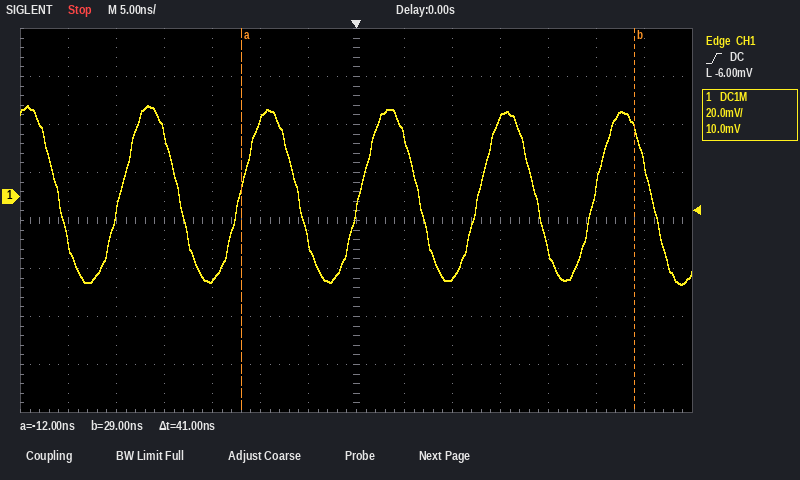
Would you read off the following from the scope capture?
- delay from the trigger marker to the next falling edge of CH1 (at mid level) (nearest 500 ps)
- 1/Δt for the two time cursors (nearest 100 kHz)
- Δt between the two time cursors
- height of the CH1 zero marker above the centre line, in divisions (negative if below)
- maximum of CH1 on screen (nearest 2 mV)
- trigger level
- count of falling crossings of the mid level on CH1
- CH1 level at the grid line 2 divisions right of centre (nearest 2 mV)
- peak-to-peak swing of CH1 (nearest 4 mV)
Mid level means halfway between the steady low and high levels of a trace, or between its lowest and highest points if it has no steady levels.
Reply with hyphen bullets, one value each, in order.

- 6.5 ns
- 24.4 MHz
- 41 ns
- +0.5 div
- 38 mV
- -6.00 mV
- 6
- -34 mV
- 76 mV
